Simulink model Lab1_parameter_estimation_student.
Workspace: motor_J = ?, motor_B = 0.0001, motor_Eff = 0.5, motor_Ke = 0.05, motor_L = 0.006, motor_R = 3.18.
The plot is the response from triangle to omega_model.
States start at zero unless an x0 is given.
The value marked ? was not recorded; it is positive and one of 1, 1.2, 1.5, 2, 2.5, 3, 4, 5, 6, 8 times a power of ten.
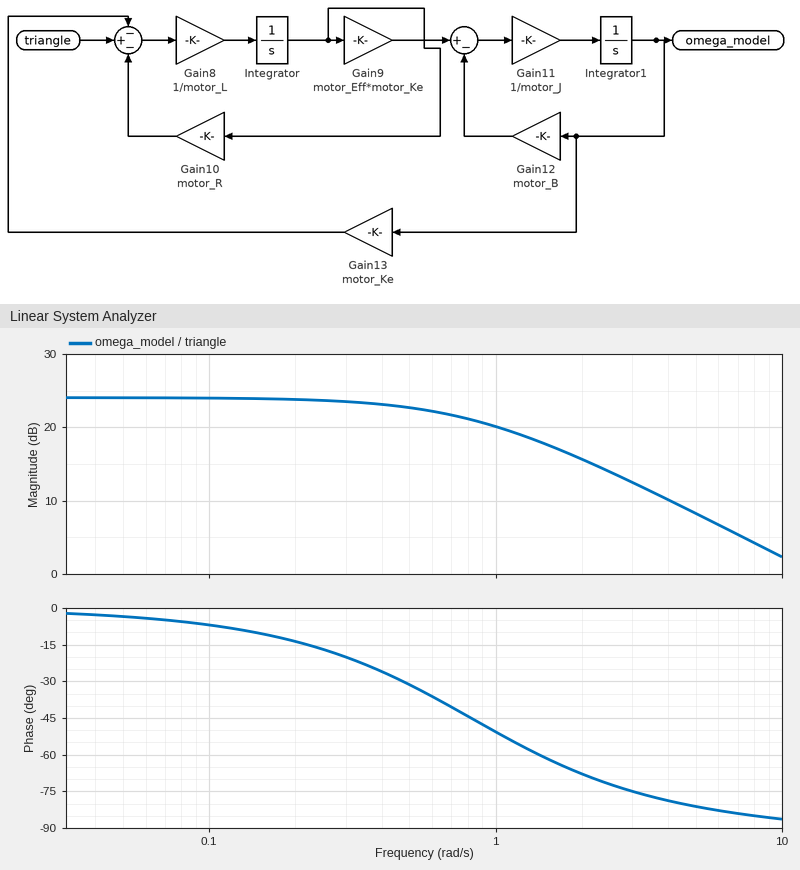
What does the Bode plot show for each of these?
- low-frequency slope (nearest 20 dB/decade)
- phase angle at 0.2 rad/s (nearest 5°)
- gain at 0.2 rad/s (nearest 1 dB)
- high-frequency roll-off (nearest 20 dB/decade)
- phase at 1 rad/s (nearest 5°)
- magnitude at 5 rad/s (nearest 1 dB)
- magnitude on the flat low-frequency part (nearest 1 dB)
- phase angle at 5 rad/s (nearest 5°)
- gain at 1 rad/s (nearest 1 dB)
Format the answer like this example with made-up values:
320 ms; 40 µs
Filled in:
0 dB/decade; -15°; 24 dB; -20 dB/decade; -50°; 8 dB; 24 dB; -80°; 20 dB
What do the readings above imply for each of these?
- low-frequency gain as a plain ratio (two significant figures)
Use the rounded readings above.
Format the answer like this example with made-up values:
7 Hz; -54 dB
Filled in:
16
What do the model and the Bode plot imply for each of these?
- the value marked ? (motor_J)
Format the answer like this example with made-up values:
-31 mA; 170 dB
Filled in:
0.0006
